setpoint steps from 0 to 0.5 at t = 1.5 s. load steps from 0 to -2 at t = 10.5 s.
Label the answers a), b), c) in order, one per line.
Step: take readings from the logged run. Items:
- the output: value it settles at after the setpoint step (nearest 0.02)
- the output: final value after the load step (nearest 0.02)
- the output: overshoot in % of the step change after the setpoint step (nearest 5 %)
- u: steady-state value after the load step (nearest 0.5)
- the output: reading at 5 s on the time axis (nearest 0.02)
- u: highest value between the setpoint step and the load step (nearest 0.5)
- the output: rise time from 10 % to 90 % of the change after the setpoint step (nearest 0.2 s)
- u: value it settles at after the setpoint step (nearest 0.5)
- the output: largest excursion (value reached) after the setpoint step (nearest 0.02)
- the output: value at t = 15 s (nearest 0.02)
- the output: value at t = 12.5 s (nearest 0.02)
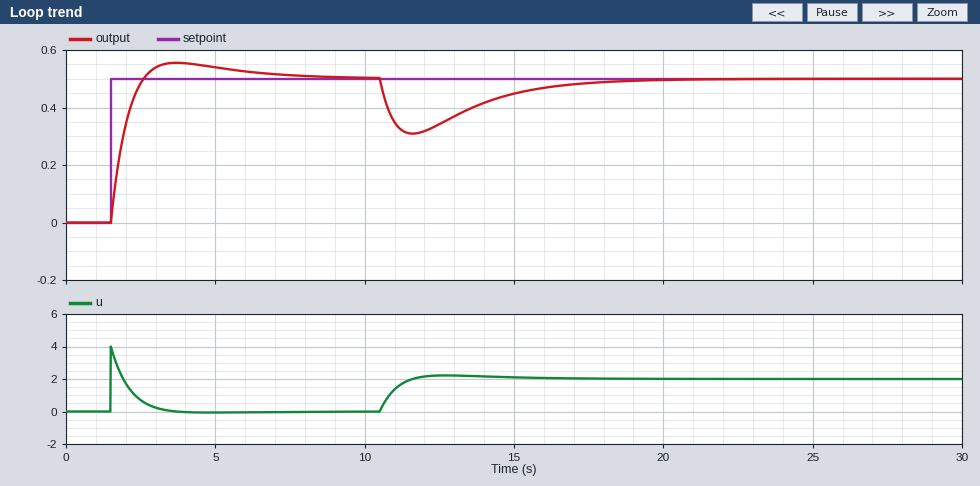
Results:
a) 0.50
b) 0.50
c) 10 %
d) 2.0
e) 0.54
f) 4.0
g) 0.8 s
h) 0.0
i) 0.56
j) 0.44
k) 0.34
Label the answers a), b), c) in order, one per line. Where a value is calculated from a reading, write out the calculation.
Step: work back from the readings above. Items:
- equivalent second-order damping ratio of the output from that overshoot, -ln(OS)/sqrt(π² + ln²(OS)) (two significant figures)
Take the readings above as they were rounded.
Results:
a) ln(0.1) = -2.303; 2.303 / sqrt(9.870 + 5.302) = 0.59
